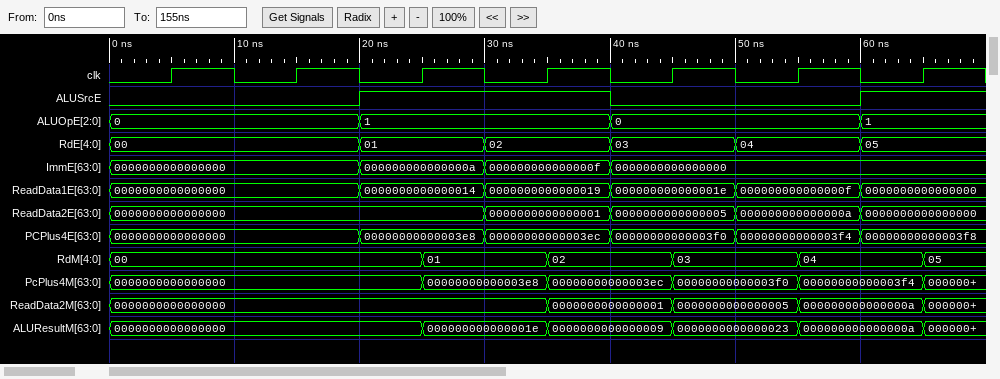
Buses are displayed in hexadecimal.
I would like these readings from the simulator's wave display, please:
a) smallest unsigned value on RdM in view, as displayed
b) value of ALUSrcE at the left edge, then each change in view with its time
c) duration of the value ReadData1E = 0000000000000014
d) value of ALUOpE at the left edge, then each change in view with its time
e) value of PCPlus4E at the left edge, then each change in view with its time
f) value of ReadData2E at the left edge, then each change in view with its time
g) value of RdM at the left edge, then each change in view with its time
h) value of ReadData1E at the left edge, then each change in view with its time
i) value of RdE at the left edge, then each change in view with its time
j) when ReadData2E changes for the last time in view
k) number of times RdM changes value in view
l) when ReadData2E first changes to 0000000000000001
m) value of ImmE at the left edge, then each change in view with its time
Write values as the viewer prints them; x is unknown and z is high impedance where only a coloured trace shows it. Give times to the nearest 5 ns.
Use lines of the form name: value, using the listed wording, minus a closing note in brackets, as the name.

smallest unsigned value on RdM in view, as displayed: 00
value of ALUSrcE at the left edge, then each change in view with its time: 0, 1 at 20 ns, 0 at 40 ns, 1 at 60 ns
duration of the value ReadData1E = 0000000000000014: 10 ns
value of ALUOpE at the left edge, then each change in view with its time: 0, 1 at 20 ns, 0 at 40 ns, 1 at 60 ns
value of PCPlus4E at the left edge, then each change in view with its time: 0000000000000000, 00000000000003e8 at 20 ns, 00000000000003ec at 30 ns, 00000000000003f0 at 40 ns, 00000000000003f4 at 50 ns, 00000000000003f8 at 60 ns
value of ReadData2E at the left edge, then each change in view with its time: 0000000000000000, 0000000000000001 at 30 ns, 0000000000000005 at 40 ns, 000000000000000a at 50 ns, 0000000000000000 at 60 ns
value of RdM at the left edge, then each change in view with its time: 00, 01 at 25 ns, 02 at 35 ns, 03 at 45 ns, 04 at 55 ns, 05 at 65 ns
value of ReadData1E at the left edge, then each change in view with its time: 0000000000000000, 0000000000000014 at 20 ns, 0000000000000019 at 30 ns, 000000000000001e at 40 ns, 000000000000000f at 50 ns, 0000000000000000 at 60 ns
value of RdE at the left edge, then each change in view with its time: 00, 01 at 20 ns, 02 at 30 ns, 03 at 40 ns, 04 at 50 ns, 05 at 60 ns
when ReadData2E changes for the last time in view: 60 ns
number of times RdM changes value in view: 5
when ReadData2E first changes to 0000000000000001: 30 ns
value of ImmE at the left edge, then each change in view with its time: 0000000000000000, 000000000000000a at 20 ns, 000000000000000f at 30 ns, 0000000000000000 at 40 ns
